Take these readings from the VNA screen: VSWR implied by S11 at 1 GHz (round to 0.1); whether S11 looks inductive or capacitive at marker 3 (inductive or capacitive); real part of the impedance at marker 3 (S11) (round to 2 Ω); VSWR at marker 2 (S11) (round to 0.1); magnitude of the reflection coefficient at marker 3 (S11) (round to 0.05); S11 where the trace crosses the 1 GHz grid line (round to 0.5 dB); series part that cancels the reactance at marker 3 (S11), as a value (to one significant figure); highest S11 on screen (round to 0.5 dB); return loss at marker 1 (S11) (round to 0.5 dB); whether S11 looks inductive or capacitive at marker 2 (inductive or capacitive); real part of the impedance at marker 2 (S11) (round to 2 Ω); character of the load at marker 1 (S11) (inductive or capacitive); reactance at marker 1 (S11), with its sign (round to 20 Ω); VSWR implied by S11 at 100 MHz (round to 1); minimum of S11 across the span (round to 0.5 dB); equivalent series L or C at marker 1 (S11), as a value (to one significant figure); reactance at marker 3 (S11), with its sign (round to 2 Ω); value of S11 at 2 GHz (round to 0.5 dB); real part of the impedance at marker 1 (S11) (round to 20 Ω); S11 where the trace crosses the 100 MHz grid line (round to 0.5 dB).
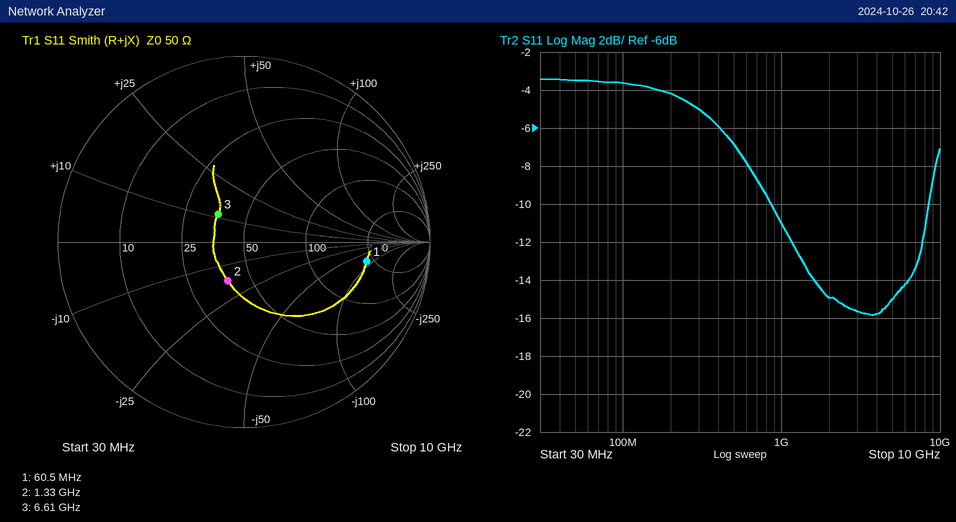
1.8
inductive
36 Ω
1.6
0.20
-11.0 dB
2 pF
-3.5 dB
3.5 dB
capacitive
38 Ω
capacitive
-80 Ω
5
-16.0 dB
30 pF
+12 Ω
-15.0 dB
220 Ω
-3.5 dB
